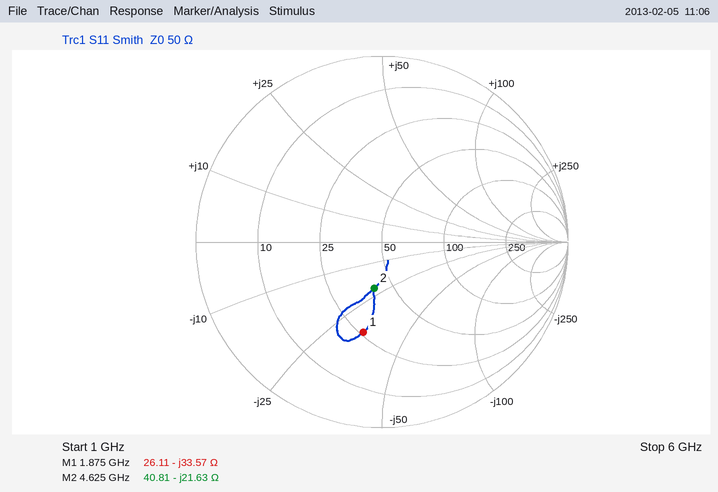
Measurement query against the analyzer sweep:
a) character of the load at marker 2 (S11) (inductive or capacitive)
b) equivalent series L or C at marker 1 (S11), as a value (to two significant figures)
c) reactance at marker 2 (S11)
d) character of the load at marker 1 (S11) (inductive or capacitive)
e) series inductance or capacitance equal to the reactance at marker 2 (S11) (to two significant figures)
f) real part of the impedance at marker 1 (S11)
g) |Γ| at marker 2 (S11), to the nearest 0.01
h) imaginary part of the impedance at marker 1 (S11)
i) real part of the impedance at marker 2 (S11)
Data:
capacitive
2.5 pF
-21.63 Ω
capacitive
1.6 pF
26.11 Ω
0.25
-33.57 Ω
40.81 Ω
